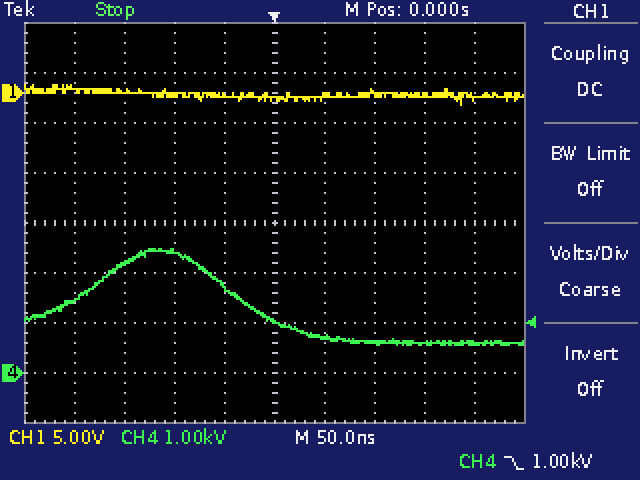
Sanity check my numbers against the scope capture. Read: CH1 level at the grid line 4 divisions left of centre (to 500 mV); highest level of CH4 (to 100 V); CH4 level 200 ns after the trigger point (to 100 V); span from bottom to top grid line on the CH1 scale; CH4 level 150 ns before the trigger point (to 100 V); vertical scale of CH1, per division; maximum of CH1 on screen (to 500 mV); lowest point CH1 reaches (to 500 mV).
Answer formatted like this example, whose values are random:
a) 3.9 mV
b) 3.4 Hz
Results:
a) 500 mV
b) 2.5 kV
c) 600 V
d) 40 V
e) 2.2 kV
f) 5 V
g) 1.0 V
h) -1.0 V
